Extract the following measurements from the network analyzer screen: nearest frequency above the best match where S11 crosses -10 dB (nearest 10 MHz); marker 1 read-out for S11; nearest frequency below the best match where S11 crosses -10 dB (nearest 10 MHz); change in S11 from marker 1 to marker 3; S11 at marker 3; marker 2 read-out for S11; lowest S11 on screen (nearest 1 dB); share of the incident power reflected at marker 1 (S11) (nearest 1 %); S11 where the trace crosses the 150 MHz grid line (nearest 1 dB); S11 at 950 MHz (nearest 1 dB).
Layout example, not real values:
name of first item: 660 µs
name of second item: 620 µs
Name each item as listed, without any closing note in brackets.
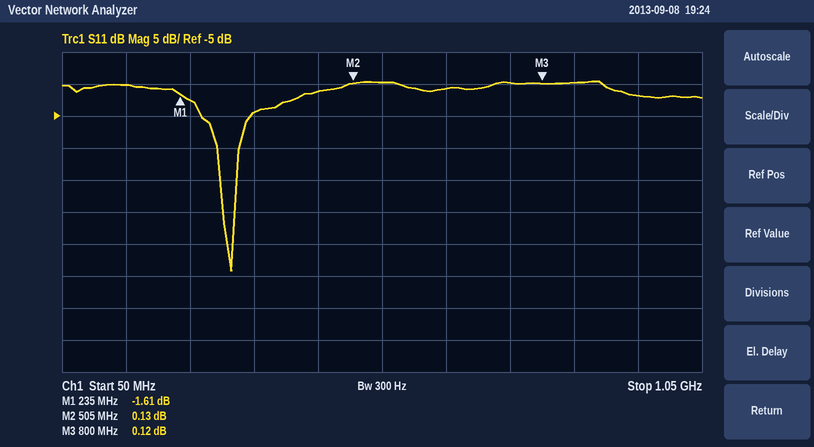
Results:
nearest frequency above the best match where S11 crosses -10 dB: 330 MHz
marker 1 read-out for S11: -1.61 dB
nearest frequency below the best match where S11 crosses -10 dB: 290 MHz
change in S11 from marker 1 to marker 3: 1.73 dB
S11 at marker 3: 0.12 dB
marker 2 read-out for S11: 0.13 dB
lowest S11 on screen: -29 dB
share of the incident power reflected at marker 1 (S11): 69 %
S11 where the trace crosses the 150 MHz grid line: 0 dB
S11 at 950 MHz: -2 dB
